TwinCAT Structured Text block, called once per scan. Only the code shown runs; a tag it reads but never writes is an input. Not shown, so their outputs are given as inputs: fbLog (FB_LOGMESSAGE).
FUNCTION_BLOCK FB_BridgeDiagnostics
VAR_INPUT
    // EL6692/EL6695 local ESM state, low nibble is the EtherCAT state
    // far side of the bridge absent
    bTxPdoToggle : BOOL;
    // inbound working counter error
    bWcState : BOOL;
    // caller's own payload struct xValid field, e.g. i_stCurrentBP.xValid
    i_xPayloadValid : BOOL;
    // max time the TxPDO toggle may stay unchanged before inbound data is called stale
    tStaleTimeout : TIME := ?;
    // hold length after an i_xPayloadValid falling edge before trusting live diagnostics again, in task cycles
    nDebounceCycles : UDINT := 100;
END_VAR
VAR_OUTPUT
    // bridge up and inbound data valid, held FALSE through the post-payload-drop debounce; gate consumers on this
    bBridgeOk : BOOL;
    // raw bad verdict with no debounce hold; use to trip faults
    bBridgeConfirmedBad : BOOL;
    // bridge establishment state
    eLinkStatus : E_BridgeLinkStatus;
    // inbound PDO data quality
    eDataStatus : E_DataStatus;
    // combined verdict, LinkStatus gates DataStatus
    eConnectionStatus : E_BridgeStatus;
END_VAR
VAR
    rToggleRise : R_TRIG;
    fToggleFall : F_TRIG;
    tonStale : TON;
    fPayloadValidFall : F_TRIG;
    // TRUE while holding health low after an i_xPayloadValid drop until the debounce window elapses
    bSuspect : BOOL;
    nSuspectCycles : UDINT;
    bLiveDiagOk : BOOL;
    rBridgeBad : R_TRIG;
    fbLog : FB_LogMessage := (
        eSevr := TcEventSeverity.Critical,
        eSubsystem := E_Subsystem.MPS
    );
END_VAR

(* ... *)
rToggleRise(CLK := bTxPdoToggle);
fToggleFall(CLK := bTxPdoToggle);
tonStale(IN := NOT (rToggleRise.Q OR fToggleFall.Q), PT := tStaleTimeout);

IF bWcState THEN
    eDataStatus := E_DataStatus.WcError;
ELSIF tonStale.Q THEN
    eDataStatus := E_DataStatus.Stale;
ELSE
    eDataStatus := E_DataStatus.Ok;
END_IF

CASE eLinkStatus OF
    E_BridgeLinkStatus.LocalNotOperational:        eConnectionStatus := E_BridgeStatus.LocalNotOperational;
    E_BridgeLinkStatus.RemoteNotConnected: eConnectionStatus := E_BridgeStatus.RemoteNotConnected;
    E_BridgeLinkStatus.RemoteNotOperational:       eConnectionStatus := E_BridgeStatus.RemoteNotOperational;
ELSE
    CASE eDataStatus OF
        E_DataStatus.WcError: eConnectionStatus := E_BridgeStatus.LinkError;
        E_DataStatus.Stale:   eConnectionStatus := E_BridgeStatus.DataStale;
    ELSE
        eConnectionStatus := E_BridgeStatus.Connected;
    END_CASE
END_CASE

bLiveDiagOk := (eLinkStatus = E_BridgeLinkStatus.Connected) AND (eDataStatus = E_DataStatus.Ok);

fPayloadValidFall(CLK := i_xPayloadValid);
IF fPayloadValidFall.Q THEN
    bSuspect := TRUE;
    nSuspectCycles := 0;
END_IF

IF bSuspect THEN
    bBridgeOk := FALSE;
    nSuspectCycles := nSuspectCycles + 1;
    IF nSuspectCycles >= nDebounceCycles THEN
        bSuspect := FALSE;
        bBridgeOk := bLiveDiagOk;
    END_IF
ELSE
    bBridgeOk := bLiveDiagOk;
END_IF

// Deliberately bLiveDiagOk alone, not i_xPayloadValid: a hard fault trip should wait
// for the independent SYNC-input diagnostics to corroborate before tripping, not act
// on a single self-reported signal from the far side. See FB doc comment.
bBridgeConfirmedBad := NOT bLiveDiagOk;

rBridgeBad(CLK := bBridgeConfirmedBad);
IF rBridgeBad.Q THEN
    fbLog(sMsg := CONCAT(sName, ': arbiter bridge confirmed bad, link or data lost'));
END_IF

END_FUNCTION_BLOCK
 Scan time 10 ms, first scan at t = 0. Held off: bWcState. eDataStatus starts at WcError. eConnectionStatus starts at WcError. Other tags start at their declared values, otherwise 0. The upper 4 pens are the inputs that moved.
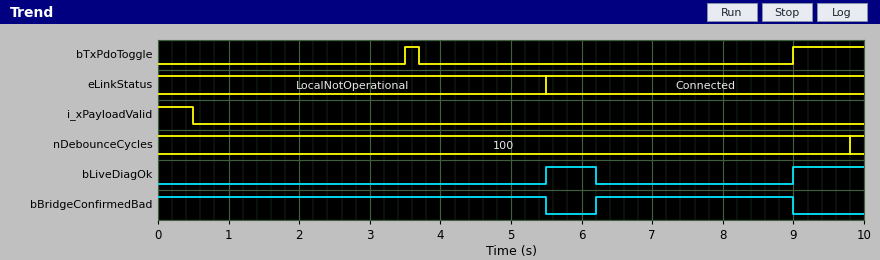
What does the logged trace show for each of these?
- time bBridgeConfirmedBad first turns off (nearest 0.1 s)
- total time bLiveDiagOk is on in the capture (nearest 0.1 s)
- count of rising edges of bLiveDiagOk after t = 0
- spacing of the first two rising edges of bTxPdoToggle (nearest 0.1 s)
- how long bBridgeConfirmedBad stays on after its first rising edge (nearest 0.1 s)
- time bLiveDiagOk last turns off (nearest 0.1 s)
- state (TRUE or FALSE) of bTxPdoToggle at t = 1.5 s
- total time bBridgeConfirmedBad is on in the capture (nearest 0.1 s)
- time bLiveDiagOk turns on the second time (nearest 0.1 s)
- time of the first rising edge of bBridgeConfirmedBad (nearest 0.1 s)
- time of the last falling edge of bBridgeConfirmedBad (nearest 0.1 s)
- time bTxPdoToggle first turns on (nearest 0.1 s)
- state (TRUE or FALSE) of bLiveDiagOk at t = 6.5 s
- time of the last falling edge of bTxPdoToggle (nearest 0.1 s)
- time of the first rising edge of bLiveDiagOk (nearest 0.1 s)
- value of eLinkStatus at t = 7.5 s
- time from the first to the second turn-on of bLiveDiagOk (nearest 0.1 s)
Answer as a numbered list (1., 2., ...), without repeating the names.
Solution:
1. 5.5 s
2. 1.7 s
3. 2
4. 5.5 s
5. 2.8 s
6. 6.2 s
7. FALSE
8. 8.3 s
9. 9.0 s
10. 6.2 s
11. 9.0 s
12. 3.5 s
13. FALSE
14. 3.7 s
15. 5.5 s
16. Connected
17. 3.5 s
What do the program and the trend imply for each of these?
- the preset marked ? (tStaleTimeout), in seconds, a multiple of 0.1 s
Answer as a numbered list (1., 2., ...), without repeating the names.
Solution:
1. 2.5 s
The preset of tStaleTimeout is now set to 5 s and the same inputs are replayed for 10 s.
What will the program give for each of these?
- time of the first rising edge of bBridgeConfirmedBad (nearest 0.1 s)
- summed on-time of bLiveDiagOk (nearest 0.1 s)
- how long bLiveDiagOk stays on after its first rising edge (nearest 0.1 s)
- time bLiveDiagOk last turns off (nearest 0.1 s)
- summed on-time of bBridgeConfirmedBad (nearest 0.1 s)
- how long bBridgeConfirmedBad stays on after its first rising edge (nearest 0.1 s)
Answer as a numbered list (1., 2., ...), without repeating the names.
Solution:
1. 8.7 s
2. 4.2 s
3. 3.2 s
4. 8.7 s
5. 5.8 s
6. 0.3 s
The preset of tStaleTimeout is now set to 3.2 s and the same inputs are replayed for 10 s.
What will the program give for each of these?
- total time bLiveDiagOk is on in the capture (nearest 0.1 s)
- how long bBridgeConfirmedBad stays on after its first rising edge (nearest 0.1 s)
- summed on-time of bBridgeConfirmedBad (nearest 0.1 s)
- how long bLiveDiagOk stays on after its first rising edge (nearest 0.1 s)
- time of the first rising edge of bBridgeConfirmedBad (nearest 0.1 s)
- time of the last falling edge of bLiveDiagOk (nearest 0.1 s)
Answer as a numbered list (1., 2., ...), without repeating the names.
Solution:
1. 2.4 s
2. 2.1 s
3. 7.6 s
4. 1.4 s
5. 6.9 s
6. 6.9 s
